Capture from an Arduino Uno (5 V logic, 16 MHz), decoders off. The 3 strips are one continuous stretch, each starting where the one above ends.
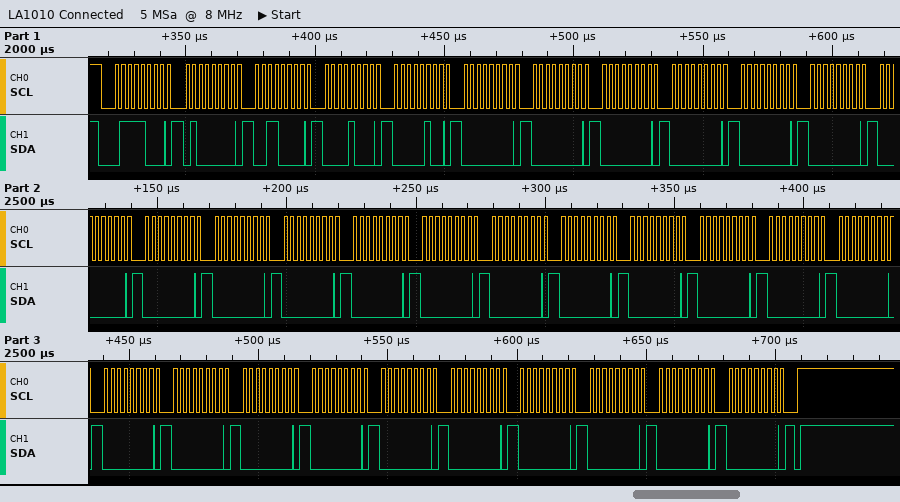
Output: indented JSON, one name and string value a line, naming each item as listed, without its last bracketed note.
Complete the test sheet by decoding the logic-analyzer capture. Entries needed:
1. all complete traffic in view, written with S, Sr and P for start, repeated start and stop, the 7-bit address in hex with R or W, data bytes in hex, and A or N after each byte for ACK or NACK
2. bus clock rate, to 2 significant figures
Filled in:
{
  "all complete traffic in view, written with S, Sr and P for start, repeated start and stop, the 7-bit address in hex with R or W, data bytes in hex, and A or N after each byte for ACK or NACK": "S 3CW A 40 A 30 A 08 A 04 A 00 A 00 A 00 A 00 A 00 A 00 A 00 A 00 A 00 A 00 A 00 A 00 A 00 A 00 A 00 A 00 A 00 A 00 A 00 A 00 A 00 A 00 A 00 A 00 A 00 A 00 A 00 A 00 A P",
  "bus clock rate, to 2 significant figures": "400 kHz"
}
